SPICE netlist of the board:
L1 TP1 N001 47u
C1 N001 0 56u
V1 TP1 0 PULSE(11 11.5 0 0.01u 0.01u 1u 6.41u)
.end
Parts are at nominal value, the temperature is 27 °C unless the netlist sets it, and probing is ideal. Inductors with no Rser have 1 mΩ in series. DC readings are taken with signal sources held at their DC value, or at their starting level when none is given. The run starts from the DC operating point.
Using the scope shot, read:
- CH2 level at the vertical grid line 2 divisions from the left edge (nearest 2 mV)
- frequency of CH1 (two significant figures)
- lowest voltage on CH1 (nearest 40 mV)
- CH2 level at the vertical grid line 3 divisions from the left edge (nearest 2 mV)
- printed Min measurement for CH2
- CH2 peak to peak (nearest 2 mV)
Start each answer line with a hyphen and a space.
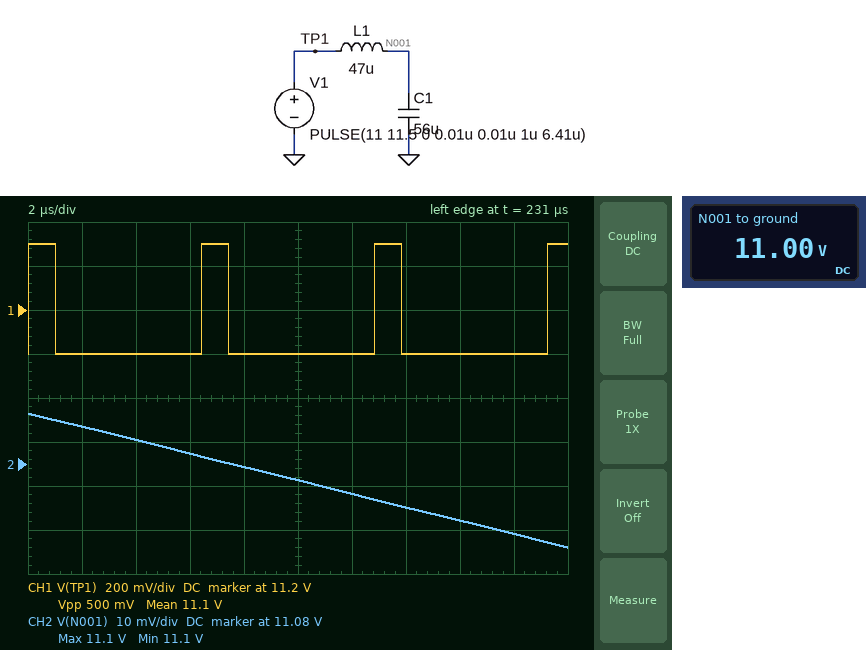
- 11.086 V
- 160 kHz
- 11.00 V
- 11.082 V
- 11.1 V
- 30 mV
